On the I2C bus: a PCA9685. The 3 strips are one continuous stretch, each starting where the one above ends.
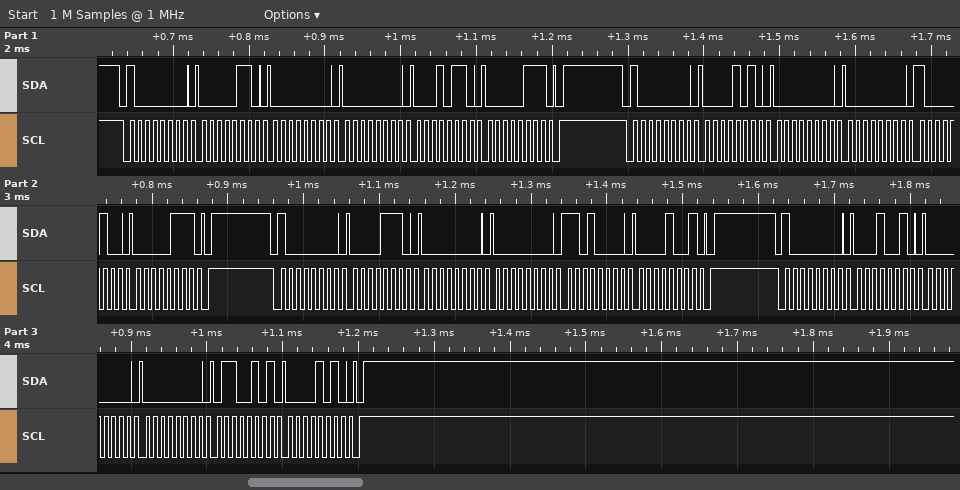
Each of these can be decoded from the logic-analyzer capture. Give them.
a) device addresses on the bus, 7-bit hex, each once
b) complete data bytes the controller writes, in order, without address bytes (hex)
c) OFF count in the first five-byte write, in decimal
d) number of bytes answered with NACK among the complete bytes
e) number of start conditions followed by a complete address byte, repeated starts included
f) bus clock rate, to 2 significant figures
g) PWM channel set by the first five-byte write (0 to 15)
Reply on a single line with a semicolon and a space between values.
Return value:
0x40; 06 00 00 16 07 0A 00 00 84 07 0E 00 00 D0 09 12 00 00 65 0A; 1814; 0; 4; 100 kHz; 0
